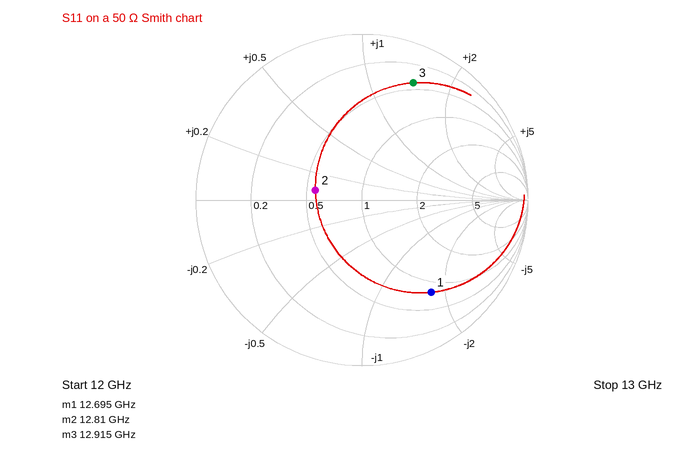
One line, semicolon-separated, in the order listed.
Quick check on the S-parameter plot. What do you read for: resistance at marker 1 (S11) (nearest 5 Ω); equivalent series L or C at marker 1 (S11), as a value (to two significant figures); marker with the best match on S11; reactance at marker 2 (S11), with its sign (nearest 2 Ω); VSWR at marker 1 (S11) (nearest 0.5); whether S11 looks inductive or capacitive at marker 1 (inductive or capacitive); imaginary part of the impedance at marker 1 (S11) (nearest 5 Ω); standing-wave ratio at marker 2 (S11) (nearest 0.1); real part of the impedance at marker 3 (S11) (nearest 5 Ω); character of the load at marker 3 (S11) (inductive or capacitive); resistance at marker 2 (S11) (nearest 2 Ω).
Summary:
40 Ω; 150 fF; marker 2; +4 Ω; 5.5; capacitive; -85 Ω; 1.8; 20 Ω; inductive; 28 Ω
